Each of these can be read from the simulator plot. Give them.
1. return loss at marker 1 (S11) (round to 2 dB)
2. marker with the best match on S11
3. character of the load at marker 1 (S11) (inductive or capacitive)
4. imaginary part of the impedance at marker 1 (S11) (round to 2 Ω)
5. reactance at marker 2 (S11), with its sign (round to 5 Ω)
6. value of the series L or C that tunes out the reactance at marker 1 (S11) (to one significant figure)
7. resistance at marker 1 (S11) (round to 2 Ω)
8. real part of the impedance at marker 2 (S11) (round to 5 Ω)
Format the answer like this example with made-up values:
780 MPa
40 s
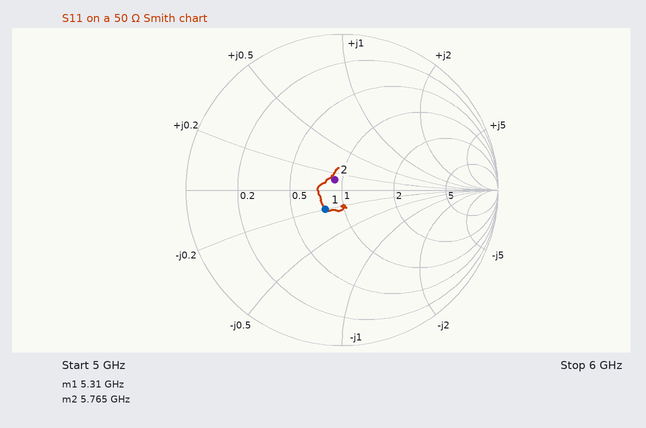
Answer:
16 dB
marker 2
capacitive
-10 Ω
+5 Ω
300 pH
40 Ω
45 Ω
